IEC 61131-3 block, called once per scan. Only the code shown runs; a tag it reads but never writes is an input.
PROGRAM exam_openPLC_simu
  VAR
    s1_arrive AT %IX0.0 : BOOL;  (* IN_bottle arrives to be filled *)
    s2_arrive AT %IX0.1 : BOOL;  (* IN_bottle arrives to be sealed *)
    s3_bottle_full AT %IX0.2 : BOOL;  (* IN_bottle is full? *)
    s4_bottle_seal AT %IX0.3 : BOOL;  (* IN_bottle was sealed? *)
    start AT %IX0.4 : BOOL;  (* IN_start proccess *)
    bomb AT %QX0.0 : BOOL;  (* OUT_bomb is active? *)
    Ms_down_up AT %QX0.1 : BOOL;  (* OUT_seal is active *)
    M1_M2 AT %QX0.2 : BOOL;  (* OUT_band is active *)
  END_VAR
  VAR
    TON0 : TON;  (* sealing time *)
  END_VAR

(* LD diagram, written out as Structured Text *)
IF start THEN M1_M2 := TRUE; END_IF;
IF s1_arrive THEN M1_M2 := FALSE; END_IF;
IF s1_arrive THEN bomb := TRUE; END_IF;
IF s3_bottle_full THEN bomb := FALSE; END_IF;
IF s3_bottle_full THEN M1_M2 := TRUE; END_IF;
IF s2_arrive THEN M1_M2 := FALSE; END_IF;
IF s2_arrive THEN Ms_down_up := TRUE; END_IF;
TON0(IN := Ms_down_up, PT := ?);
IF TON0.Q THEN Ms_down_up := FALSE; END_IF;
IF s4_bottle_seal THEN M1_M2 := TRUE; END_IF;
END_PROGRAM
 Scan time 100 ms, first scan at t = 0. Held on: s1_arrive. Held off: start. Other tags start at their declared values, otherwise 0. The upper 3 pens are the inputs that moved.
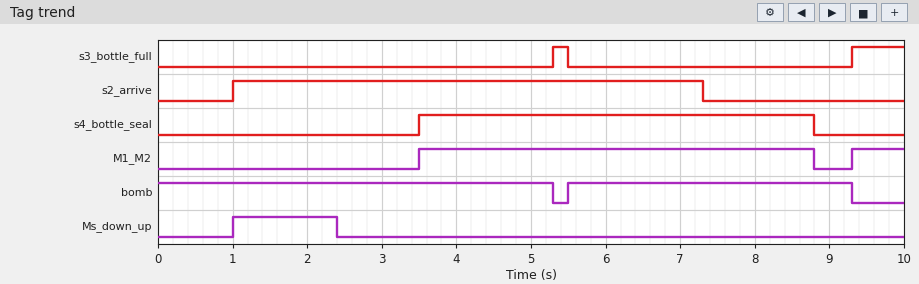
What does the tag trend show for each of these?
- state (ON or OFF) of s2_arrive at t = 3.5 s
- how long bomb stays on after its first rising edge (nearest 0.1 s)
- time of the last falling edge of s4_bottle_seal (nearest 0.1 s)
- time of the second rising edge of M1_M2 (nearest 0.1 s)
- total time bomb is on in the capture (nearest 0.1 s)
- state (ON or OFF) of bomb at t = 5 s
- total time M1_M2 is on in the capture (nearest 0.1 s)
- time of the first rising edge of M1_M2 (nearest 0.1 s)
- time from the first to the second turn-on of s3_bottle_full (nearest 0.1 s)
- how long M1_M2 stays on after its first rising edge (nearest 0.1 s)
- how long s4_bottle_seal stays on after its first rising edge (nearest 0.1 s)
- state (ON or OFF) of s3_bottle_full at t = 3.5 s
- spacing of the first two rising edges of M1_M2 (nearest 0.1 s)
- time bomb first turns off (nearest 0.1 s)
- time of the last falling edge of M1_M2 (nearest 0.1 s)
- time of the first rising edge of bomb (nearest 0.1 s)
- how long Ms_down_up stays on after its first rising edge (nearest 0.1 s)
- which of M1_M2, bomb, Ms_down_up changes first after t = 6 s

ON
3.8 s
8.8 s
9.3 s
9.1 s
ON
6.0 s
3.5 s
4.0 s
5.3 s
5.3 s
OFF
5.8 s
5.3 s
8.8 s
5.5 s
1.4 s
M1_M2
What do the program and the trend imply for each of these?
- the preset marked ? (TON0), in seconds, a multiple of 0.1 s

1.4 s
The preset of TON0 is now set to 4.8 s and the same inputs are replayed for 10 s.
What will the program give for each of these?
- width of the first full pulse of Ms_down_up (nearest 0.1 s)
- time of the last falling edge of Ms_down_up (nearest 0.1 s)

4.8 s
5.8 s
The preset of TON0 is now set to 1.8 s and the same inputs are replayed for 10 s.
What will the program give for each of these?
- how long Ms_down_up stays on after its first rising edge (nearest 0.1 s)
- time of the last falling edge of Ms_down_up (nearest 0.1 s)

1.8 s
2.8 s
